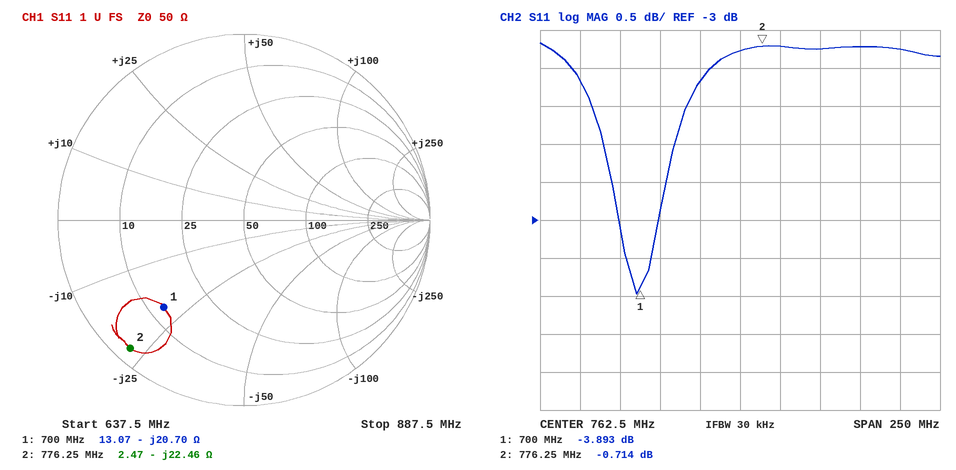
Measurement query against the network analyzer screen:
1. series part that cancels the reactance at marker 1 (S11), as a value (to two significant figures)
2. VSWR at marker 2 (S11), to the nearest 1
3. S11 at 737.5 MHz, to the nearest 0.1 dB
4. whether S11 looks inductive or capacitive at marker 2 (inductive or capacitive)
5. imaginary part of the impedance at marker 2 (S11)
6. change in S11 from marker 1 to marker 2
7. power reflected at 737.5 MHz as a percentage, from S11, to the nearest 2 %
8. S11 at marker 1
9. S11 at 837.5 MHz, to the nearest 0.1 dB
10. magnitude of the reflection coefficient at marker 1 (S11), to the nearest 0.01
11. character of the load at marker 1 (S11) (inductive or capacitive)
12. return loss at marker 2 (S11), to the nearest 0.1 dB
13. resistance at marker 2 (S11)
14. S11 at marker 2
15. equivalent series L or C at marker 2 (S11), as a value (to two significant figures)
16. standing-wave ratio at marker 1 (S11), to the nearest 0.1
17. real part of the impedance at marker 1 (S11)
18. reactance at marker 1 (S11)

4.7 nH
24
-1.2 dB
capacitive
-22.46 Ω
3.179 dB
76 %
-3.893 dB
-0.7 dB
0.64
capacitive
0.7 dB
2.47 Ω
-0.714 dB
9.1 pF
4.5
13.07 Ω
-20.70 Ω
